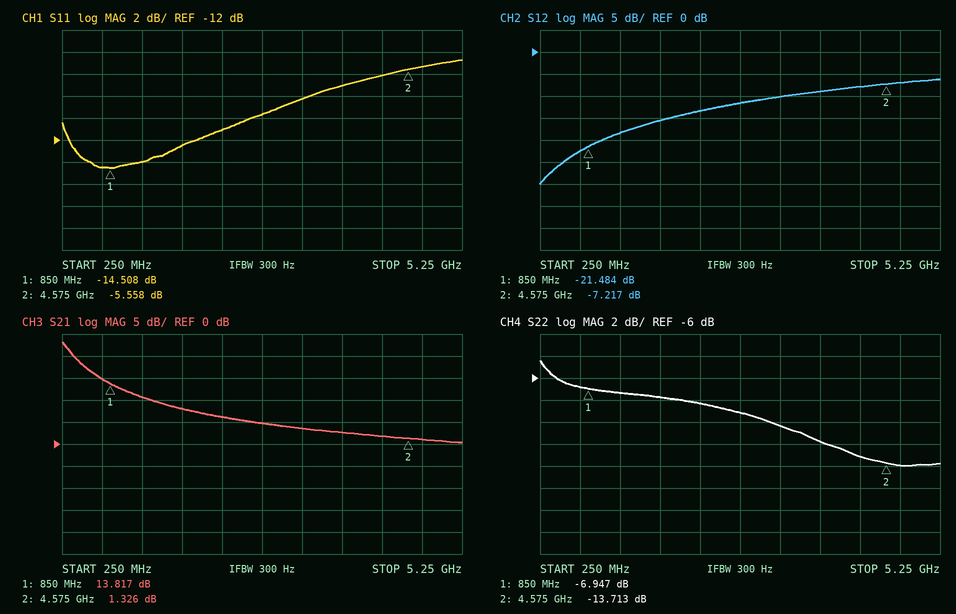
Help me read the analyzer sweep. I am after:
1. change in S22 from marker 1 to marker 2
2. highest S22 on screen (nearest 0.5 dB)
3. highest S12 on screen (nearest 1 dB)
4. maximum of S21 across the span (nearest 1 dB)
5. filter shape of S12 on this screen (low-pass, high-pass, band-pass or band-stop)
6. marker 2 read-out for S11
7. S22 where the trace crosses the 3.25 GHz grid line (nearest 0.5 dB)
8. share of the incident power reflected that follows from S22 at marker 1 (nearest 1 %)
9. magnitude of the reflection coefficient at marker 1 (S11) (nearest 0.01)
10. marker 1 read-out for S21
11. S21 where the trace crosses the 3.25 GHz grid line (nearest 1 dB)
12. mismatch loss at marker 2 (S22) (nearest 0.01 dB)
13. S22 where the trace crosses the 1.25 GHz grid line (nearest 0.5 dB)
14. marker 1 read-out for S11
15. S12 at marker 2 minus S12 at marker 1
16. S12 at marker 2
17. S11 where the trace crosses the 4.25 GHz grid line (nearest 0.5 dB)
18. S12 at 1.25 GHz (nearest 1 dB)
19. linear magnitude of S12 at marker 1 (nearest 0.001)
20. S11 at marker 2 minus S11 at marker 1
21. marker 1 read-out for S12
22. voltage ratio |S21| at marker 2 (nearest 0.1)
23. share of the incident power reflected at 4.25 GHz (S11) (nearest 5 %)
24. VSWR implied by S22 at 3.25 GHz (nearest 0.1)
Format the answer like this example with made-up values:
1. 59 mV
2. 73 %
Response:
1. -6.766 dB
2. -4.5 dB
3. -6 dB
4. 23 dB
5. high-pass
6. -5.558 dB
7. -10.5 dB
8. 20 %
9. 0.19
10. 13.817 dB
11. 4 dB
12. 0.19 dB
13. -7.5 dB
14. -14.508 dB
15. 14.267 dB
16. -7.217 dB
17. -6.0 dB
18. -18 dB
19. 0.084
20. 8.950 dB
21. -21.484 dB
22. 1.2
23. 25 %
24. 1.9
